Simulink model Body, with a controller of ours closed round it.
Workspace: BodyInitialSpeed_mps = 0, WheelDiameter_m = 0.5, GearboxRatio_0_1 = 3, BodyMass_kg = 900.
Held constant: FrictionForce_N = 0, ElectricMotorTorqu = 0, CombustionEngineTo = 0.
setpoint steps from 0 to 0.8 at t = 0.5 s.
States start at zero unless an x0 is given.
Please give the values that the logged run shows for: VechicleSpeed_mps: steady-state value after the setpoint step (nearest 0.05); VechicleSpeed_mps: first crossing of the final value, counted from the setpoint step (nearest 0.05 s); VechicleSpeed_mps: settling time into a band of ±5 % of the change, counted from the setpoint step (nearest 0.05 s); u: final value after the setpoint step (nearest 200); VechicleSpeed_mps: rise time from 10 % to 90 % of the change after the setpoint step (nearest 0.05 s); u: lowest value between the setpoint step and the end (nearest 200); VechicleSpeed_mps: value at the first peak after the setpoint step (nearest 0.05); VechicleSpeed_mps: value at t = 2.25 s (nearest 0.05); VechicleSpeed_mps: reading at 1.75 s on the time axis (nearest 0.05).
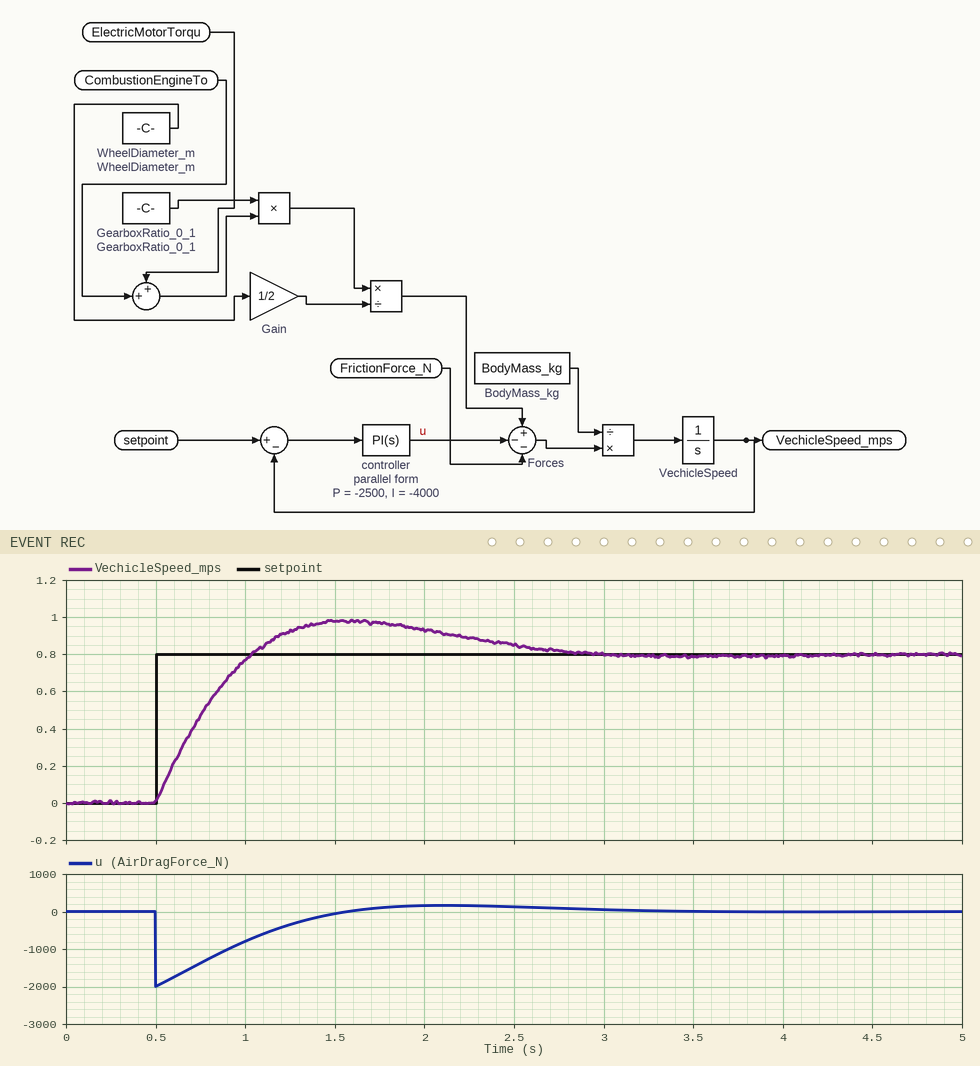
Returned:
0.80
0.55 s
2.05 s
0
0.40 s
-2000
1.00
0.90
0.95
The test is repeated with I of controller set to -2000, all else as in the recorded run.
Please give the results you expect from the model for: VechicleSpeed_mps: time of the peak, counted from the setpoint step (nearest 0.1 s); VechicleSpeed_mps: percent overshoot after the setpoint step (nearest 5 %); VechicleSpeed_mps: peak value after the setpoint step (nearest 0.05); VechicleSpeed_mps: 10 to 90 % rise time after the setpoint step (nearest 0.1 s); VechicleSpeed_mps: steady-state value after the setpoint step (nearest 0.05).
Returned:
1.4 s
15 %
0.90
0.5 s
0.80
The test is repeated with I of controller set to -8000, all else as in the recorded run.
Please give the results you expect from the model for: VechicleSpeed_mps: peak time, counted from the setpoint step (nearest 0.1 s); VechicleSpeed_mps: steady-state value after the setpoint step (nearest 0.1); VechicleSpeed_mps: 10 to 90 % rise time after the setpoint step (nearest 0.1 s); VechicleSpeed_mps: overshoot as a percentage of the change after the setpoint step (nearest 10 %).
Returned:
0.8 s
0.8
0.3 s
30 %
